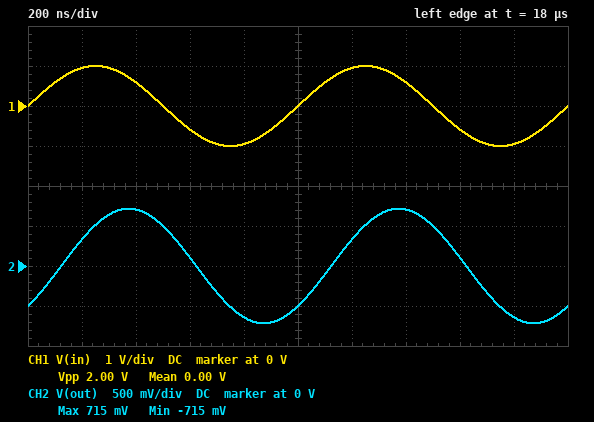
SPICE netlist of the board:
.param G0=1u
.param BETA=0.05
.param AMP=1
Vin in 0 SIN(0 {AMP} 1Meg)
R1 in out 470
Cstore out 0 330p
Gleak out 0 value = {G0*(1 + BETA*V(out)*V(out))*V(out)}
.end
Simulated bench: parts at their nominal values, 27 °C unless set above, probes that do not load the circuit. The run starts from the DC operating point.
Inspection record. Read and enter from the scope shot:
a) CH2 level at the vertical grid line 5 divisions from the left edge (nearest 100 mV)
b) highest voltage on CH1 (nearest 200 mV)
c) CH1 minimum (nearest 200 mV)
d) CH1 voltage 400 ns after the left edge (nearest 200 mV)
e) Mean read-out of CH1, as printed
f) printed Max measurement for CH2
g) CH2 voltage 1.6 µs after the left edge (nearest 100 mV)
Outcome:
-500 mV
1.0 V
-1.0 V
600 mV
0.00 V
715 mV
100 mV
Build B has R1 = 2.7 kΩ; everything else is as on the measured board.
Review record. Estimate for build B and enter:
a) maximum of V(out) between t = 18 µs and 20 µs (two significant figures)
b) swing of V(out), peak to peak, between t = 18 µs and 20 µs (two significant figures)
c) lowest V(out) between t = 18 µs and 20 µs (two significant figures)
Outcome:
180 mV
350 mV
-180 mV
